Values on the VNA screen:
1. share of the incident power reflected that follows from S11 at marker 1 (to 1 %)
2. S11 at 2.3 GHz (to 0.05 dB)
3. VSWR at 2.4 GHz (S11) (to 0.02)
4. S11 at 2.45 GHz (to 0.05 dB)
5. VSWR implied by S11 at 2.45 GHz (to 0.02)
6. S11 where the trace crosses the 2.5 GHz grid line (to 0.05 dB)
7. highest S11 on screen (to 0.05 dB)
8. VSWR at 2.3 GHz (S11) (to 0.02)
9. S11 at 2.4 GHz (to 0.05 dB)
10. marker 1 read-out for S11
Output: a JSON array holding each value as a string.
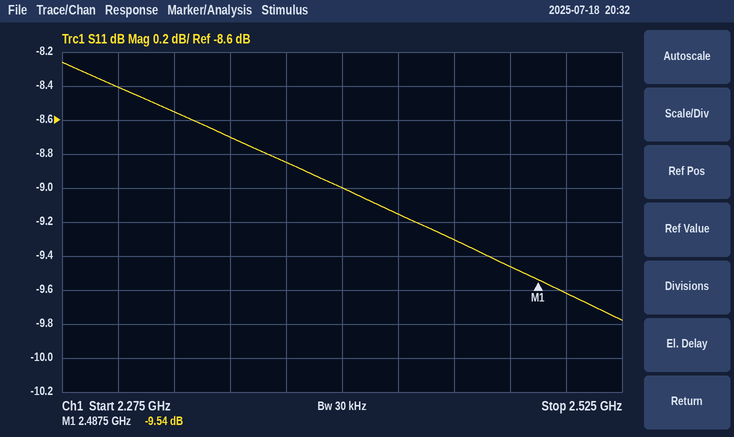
["11 %", "-8.40 dB", "2.10", "-9.30 dB", "2.04", "-9.60 dB", "-8.25 dB", "2.22", "-9.00 dB", "-9.54 dB"]
